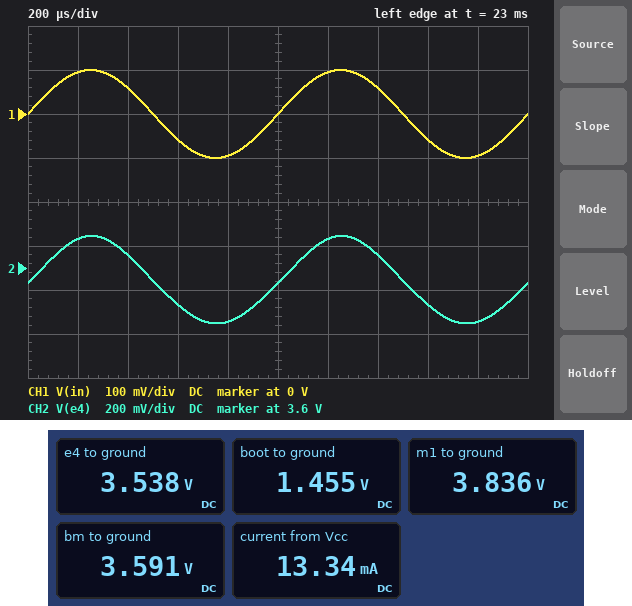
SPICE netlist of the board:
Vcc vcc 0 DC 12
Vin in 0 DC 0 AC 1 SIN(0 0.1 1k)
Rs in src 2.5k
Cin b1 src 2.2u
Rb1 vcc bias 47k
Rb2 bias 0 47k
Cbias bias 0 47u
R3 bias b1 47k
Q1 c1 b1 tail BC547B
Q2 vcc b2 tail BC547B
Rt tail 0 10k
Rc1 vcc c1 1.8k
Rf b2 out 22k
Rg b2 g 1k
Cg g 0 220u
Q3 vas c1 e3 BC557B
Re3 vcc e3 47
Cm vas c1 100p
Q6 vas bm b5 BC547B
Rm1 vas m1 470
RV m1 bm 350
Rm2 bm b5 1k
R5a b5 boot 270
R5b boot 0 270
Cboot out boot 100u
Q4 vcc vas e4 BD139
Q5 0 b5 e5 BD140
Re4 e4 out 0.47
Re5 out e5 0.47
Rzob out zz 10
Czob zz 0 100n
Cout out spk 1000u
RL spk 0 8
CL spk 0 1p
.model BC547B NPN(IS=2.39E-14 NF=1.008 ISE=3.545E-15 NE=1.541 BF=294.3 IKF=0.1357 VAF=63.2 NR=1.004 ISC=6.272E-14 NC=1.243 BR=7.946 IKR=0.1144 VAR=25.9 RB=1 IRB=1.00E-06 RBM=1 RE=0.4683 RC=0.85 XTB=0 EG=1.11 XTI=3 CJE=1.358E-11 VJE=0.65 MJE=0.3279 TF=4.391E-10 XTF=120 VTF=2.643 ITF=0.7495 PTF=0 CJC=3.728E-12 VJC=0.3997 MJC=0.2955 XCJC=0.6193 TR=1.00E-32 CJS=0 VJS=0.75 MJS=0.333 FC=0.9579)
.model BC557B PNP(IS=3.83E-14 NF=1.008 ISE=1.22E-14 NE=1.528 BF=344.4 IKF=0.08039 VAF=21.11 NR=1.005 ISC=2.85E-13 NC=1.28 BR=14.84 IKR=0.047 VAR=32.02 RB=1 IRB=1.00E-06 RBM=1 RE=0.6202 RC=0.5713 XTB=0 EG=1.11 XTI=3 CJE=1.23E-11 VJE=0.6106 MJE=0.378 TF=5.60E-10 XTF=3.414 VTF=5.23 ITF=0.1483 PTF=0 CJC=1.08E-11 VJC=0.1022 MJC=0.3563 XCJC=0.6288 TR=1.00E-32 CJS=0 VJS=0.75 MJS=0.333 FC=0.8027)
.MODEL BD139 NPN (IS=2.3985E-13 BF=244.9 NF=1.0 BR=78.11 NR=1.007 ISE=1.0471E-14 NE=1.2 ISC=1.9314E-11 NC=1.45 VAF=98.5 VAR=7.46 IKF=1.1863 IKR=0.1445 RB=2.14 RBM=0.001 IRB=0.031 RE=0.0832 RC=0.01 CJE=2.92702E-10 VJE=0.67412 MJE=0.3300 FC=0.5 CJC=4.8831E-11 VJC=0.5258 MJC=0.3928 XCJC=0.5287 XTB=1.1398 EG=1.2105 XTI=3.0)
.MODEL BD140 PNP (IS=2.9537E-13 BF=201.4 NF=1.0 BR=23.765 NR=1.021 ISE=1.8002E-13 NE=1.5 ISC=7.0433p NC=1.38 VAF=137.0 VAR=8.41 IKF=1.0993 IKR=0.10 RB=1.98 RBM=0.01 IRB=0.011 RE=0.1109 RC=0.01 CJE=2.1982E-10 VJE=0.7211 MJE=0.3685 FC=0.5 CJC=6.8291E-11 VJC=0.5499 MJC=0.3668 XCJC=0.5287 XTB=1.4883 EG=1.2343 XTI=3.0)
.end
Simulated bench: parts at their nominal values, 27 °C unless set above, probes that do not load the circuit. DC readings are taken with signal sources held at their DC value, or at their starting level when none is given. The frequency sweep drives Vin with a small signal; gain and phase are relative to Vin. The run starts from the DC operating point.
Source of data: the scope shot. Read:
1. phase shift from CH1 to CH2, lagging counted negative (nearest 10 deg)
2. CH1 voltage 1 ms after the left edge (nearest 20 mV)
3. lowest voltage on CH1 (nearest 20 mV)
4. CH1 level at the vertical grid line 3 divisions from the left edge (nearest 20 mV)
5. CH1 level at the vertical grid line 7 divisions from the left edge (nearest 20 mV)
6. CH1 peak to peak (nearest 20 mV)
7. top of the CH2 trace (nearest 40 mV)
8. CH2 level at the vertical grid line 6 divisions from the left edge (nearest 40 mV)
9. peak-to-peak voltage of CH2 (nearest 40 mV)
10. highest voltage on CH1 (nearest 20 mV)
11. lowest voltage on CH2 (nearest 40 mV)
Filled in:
0 deg
0 V
-100 mV
-60 mV
60 mV
200 mV
3.76 V
3.72 V
400 mV
100 mV
3.36 V
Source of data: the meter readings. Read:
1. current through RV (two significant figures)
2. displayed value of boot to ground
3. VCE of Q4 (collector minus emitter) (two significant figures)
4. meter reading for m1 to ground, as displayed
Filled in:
700 µA
1.455 V
8.5 V
3.836 V
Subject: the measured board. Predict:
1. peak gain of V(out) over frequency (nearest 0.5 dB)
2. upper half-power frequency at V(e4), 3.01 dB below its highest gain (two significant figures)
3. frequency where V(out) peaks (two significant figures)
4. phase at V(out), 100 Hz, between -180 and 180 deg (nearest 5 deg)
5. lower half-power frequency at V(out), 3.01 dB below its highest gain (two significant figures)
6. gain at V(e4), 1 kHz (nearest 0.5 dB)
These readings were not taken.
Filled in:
8.0 dB
3.6 kHz
17 Hz
-5 deg
6.1 Hz
5.5 dB
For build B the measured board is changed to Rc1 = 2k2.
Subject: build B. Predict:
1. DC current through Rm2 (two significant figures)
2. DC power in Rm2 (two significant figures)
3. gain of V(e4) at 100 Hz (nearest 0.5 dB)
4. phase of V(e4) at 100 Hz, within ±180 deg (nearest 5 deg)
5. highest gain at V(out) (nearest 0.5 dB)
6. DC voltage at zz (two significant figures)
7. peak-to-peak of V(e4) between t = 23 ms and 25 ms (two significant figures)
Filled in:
700 µA
490 µW
9.5 dB
0 deg
10.5 dB
5.4 V
580 mV
